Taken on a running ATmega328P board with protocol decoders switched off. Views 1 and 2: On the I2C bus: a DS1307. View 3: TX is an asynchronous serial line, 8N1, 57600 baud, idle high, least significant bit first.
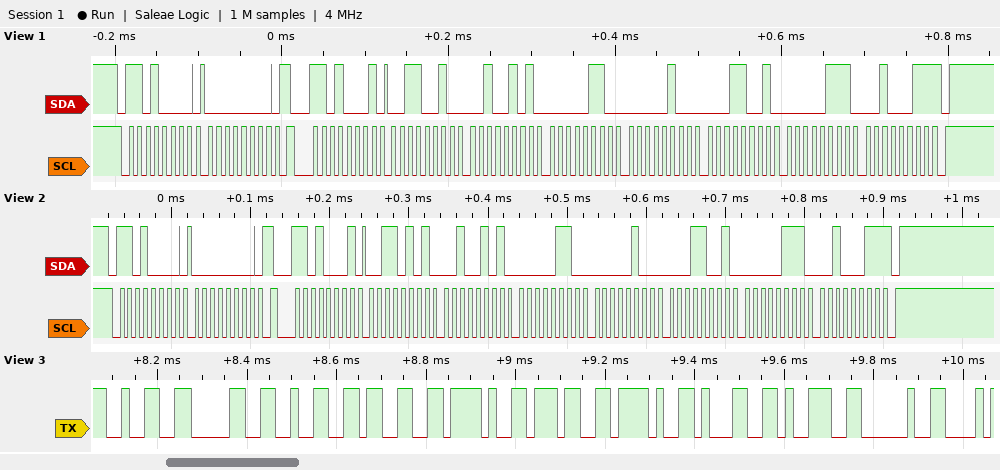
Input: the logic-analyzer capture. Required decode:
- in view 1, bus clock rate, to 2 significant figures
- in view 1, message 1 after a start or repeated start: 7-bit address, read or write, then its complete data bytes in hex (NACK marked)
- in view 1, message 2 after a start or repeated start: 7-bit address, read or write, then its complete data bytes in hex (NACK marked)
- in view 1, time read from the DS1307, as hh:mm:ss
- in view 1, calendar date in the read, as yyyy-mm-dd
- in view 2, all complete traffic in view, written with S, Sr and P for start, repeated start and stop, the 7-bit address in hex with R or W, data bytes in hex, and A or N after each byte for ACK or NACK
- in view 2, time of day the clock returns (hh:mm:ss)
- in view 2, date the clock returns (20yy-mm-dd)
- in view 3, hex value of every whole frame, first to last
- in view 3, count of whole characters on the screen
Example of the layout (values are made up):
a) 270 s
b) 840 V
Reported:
a) 100 kHz
b) 0x68 write: 00
c) 0x68 read: 32 25 06 04 19 07 23 NACK
d) 06:25:32
e) 2023-07-19
f) S 68W A 00 A Sr 68R A 35 A 25 A 06 A 04 A 19 A 07 A 23 N P
g) 06:25:35
h) 2023-07-19
i) 0x32 0x30 0x32 0x33 0x2F 0x37 0x2F 0x31 0x39 0x20
j) 10
